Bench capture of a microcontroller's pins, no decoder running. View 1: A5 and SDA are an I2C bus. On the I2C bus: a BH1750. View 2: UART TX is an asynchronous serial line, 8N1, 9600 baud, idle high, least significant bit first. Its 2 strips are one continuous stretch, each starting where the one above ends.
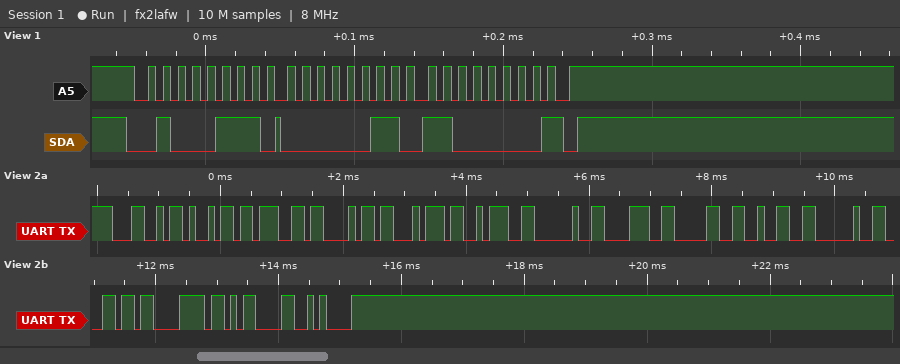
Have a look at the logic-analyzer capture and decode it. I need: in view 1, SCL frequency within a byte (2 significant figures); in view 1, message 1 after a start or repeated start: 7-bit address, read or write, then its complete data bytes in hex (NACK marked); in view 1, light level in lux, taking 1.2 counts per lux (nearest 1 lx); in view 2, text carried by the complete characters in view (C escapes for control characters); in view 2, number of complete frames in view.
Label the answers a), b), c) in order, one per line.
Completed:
a) 100 kHz
b) 0x23 read: 03 C0 NACK
c) 800 lx
d) "Light: 802 lx\r\n"
e) 15
